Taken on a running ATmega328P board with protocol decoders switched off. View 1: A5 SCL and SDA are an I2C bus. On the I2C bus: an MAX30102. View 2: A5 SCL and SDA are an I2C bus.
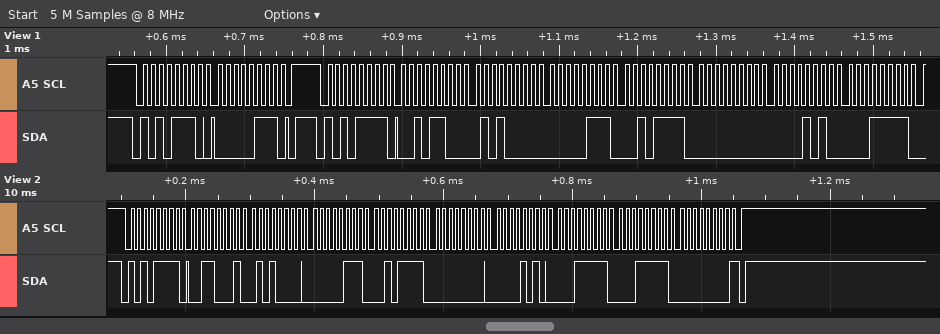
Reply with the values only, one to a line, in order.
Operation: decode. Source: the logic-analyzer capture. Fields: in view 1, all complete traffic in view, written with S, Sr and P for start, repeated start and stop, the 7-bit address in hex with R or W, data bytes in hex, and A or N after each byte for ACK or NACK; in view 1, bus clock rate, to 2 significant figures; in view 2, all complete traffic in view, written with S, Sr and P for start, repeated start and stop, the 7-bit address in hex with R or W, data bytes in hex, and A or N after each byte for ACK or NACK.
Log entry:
S 57W A 07 A P S 57R A 2C A 50 A 07 A 2F A 00 A 0A A 1F A
100 kHz
S 57R A 31 A 50 A 07 A 2F A 00 A 0A A 1F A 1F A 00 N P
